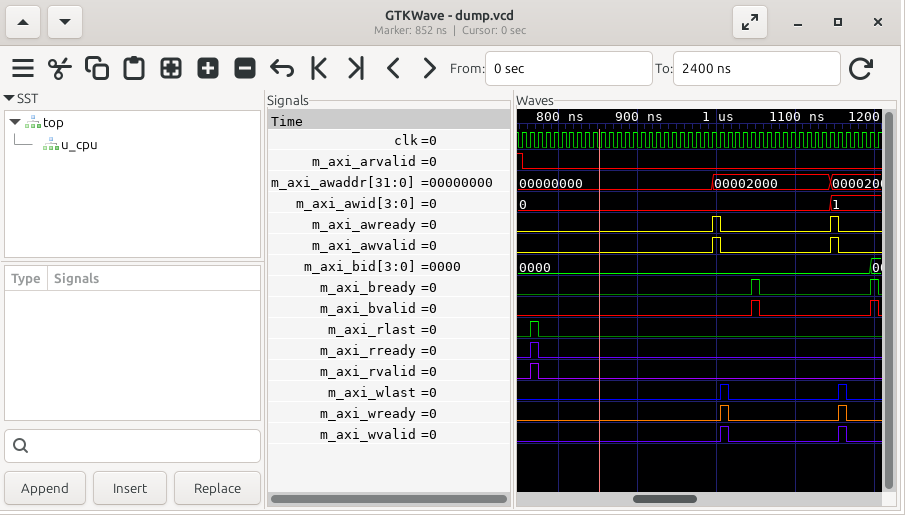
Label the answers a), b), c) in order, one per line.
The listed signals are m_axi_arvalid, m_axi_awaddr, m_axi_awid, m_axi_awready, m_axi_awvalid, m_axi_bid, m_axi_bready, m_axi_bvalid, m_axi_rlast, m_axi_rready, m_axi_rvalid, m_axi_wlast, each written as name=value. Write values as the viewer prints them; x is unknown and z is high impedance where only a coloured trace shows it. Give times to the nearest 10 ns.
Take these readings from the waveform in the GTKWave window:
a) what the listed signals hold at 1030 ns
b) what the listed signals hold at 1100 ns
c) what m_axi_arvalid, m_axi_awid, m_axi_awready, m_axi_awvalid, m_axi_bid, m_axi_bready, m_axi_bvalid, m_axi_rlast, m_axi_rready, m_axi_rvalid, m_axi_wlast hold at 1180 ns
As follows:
a) m_axi_arvalid=0, m_axi_awaddr=00002000, m_axi_awid=0, m_axi_awready=0, m_axi_awvalid=0, m_axi_bid=0000, m_axi_bready=0, m_axi_bvalid=0, m_axi_rlast=0, m_axi_rready=0, m_axi_rvalid=0, m_axi_wlast=0
b) m_axi_arvalid=0, m_axi_awaddr=00002000, m_axi_awid=0, m_axi_awready=0, m_axi_awvalid=0, m_axi_bid=0000, m_axi_bready=0, m_axi_bvalid=0, m_axi_rlast=0, m_axi_rready=0, m_axi_rvalid=0, m_axi_wlast=0
c) m_axi_arvalid=0, m_axi_awid=1, m_axi_awready=0, m_axi_awvalid=0, m_axi_bid=0000, m_axi_bready=0, m_axi_bvalid=0, m_axi_rlast=0, m_axi_rready=0, m_axi_rvalid=0, m_axi_wlast=0
